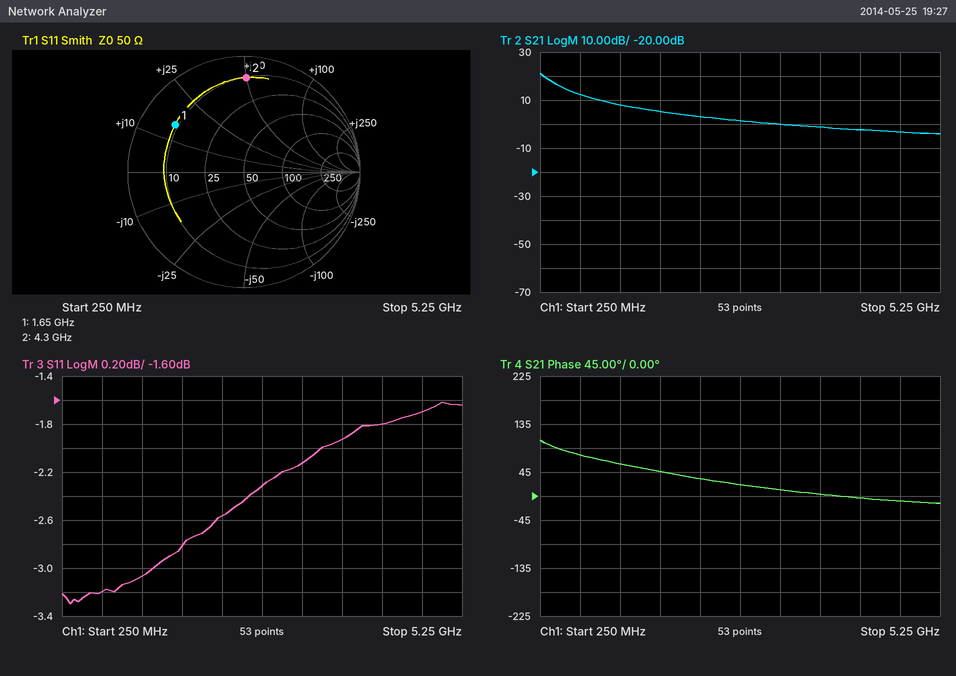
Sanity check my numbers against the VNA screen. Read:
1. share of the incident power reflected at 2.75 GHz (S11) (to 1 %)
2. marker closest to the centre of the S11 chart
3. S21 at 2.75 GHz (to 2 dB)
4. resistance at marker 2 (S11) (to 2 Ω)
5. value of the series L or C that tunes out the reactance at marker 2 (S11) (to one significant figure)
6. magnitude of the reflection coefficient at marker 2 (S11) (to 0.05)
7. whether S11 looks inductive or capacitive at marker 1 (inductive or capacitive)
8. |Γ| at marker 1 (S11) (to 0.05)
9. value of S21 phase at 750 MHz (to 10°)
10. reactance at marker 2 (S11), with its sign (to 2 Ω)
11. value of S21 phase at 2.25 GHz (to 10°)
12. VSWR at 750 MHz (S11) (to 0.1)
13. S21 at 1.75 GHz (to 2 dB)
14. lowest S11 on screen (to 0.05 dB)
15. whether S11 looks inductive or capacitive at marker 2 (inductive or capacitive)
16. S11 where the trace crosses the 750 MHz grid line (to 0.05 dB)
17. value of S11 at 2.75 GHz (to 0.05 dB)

59 %
marker 1
2 dB
10 Ω
700 fF
0.80
inductive
0.70
80°
+50 Ω
30°
5.5
6 dB
-3.30 dB
inductive
-3.20 dB
-2.30 dB
